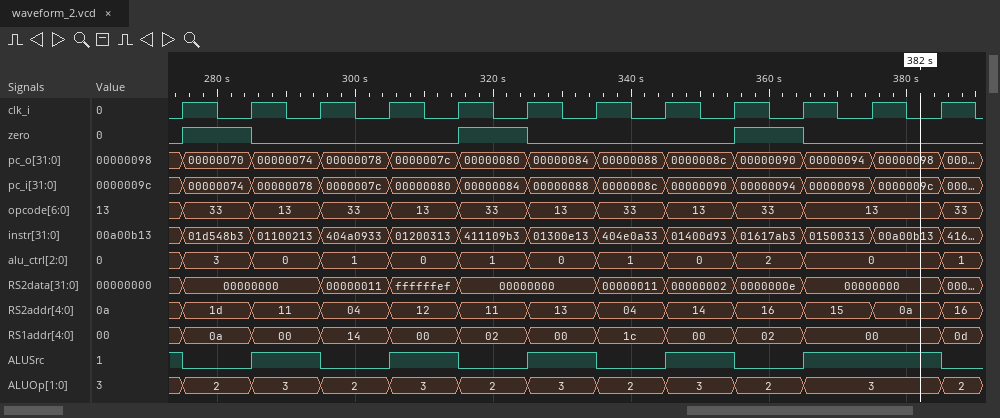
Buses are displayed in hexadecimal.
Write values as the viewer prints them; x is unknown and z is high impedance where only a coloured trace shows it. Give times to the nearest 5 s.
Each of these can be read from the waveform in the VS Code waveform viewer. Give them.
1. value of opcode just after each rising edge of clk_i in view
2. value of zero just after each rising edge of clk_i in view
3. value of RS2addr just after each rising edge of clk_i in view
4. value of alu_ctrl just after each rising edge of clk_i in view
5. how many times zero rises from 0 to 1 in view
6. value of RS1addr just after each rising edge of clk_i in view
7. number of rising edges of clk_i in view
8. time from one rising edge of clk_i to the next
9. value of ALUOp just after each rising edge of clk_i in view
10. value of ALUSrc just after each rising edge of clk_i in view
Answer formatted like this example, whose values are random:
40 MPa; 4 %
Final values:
33, 13, 33, 13, 33, 13, 33, 13, 33, 13, 13, 33; 1 0 0 0 1 0 0 0 1 0 0 0; 1d, 11, 04, 12, 11, 13, 04, 14, 16, 15, 0a, 16; 3, 0, 1, 0, 1, 0, 1, 0, 2, 0, 0, 1; 3; 0a, 00, 14, 00, 02, 00, 1c, 00, 02, 00, 00, 0d; 12; 10 s; 2, 3, 2, 3, 2, 3, 2, 3, 2, 3, 3, 2; 0 1 0 1 0 1 0 1 0 1 1 0
